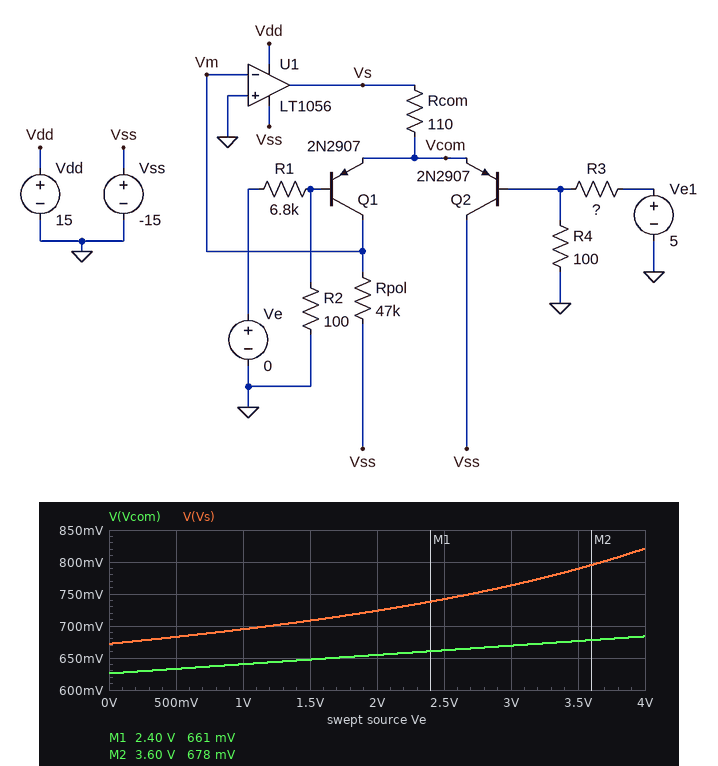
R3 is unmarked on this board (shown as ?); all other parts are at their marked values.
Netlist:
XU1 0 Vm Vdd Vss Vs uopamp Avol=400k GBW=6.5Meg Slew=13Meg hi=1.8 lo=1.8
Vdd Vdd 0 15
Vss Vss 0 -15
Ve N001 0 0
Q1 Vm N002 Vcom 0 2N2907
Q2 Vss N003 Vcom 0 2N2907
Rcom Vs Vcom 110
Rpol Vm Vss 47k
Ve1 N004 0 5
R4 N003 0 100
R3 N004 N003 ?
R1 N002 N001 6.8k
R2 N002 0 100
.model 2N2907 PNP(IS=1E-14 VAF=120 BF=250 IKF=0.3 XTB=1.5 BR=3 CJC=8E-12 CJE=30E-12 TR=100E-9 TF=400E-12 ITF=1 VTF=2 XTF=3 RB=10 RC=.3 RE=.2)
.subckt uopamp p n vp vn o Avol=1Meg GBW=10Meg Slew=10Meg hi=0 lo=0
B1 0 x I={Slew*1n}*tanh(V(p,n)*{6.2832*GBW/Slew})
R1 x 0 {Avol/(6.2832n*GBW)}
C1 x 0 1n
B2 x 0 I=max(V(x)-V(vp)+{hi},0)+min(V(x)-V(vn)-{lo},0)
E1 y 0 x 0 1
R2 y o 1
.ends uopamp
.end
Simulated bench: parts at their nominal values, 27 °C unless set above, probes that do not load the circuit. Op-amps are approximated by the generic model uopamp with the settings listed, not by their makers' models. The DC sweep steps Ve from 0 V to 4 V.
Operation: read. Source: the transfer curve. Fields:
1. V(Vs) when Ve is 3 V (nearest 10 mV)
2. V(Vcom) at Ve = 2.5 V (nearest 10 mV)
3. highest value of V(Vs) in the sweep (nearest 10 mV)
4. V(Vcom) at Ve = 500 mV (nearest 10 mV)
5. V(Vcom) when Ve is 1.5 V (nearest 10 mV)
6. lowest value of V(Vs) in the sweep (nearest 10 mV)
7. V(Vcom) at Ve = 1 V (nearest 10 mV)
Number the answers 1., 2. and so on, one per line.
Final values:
1. 760 mV
2. 660 mV
3. 820 mV
4. 630 mV
5. 650 mV
6. 670 mV
7. 640 mV
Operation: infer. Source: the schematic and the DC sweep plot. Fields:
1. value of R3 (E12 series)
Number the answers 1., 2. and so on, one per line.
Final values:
1. 15 kΩ
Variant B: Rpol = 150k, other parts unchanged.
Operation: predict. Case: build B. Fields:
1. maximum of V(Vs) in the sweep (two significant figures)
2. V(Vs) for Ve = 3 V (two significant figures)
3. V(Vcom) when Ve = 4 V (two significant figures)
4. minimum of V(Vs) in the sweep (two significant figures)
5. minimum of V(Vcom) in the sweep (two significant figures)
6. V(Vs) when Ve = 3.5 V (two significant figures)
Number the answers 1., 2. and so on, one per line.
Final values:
1. 700 mV
2. 670 mV
3. 650 mV
4. 610 mV
5. 600 mV
6. 680 mV
